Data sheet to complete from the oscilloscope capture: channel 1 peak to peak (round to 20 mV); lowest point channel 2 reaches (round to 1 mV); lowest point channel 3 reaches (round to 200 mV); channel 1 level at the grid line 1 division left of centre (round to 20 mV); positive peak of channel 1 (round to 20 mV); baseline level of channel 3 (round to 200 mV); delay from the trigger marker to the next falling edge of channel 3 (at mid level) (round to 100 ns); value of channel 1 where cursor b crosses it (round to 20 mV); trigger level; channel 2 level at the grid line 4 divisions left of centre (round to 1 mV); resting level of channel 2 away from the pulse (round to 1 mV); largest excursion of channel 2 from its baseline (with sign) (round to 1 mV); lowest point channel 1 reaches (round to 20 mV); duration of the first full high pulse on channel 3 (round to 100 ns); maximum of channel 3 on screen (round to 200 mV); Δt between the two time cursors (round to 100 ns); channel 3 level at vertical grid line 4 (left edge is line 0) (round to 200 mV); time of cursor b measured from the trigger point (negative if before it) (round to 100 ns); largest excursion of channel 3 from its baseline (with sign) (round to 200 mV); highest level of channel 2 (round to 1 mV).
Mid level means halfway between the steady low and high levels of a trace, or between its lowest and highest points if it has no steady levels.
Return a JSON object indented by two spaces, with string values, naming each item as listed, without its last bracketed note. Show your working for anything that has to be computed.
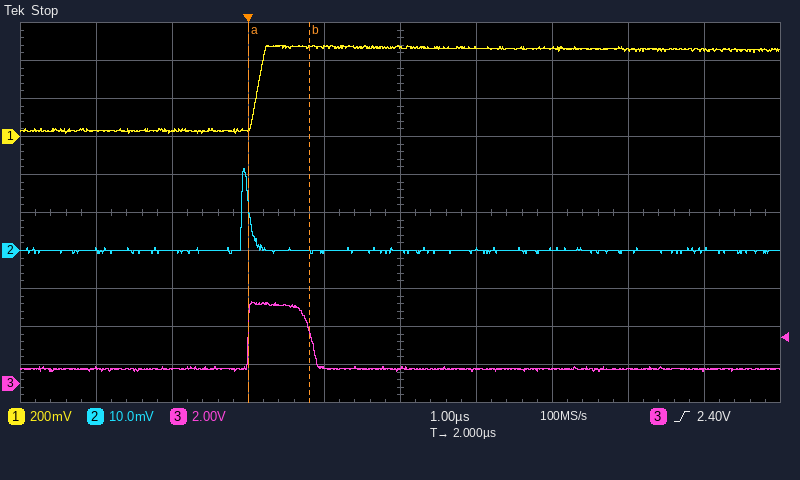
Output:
{
  "channel 1 peak to peak": "480 mV − (20 mV) = 460 mV",
  "lowest point channel 2 reaches": "-1 mV",
  "lowest point channel 3 reaches": "600 mV",
  "channel 1 level at the grid line 1 division left of centre": "480 mV",
  "positive peak of channel 1": "480 mV",
  "baseline level of channel 3": "800 mV",
  "delay from the trigger marker to the next falling edge of channel 3 (at mid level)": "800 ns",
  "value of channel 1 where cursor b crosses it": "480 mV",
  "trigger level": "2.40 V",
  "channel 2 level at the grid line 4 divisions left of centre": "0 mV",
  "resting level of channel 2 away from the pulse": "0 mV",
  "largest excursion of channel 2 from its baseline (with sign)": "22 mV − (0 mV) = +22 mV",
  "lowest point channel 1 reaches": "20 mV",
  "duration of the first full high pulse on channel 3": "800 ns",
  "maximum of channel 3 on screen": "4.4 V",
  "Δt between the two time cursors": "800 ns",
  "channel 3 level at vertical grid line 4 (left edge is line 0)": "800 mV",
  "time of cursor b measured from the trigger point (negative if before it)": "+800 ns",
  "largest excursion of channel 3 from its baseline (with sign)": "4.4 V − (800 mV) = +3.6 V",
  "highest level of channel 2": "22 mV"
}
